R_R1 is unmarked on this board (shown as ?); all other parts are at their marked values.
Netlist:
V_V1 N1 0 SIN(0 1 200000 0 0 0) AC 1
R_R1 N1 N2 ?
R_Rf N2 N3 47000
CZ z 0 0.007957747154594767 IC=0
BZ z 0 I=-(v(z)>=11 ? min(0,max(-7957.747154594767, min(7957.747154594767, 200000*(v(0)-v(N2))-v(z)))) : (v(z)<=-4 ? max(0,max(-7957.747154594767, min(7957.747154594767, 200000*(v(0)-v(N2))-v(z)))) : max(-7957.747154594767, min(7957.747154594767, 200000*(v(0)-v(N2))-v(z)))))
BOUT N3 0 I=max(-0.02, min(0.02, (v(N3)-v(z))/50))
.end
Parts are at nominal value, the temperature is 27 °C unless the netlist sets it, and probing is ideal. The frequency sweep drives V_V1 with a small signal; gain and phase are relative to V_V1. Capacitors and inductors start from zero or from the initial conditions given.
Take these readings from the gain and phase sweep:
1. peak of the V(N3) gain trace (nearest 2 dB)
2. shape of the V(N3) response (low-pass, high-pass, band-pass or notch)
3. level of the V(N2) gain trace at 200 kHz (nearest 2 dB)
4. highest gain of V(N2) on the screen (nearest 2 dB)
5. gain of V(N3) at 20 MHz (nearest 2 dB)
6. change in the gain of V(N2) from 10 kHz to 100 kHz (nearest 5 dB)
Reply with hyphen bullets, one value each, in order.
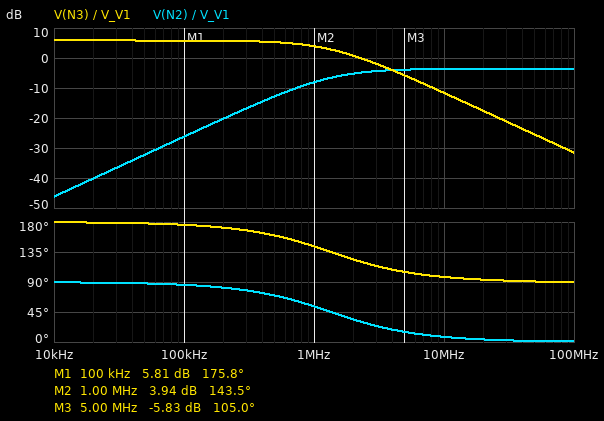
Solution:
- 6 dB
- low-pass
- -20 dB
- -4 dB
- -18 dB
- 20 dB
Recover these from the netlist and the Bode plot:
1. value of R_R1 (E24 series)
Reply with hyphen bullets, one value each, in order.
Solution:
- 24 kΩ
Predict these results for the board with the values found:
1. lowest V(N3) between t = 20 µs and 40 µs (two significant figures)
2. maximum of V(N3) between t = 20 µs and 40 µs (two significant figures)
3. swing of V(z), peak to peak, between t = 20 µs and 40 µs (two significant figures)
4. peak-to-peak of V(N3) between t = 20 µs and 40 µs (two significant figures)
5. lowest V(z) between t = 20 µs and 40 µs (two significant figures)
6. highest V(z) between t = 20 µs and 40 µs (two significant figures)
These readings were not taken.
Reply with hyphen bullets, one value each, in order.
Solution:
- -1.2 V
- 1.2 V
- 2.4 V
- 2.4 V
- -1.2 V
- 1.2 V
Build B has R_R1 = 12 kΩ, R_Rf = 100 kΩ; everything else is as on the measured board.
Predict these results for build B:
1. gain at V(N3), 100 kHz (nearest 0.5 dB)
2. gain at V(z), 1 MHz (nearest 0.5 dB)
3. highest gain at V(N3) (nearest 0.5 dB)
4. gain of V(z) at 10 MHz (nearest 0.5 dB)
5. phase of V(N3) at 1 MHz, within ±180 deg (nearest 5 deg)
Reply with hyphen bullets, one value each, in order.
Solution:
- 18.0 dB
- 10.5 dB
- 18.5 dB
- -9.0 dB
- 115 deg
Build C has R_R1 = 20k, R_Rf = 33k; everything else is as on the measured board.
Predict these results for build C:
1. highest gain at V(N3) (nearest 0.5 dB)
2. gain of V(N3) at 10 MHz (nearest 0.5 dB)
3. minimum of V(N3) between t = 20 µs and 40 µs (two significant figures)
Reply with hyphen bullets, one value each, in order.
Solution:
- 4.5 dB
- -12.0 dB
- -1.2 V
